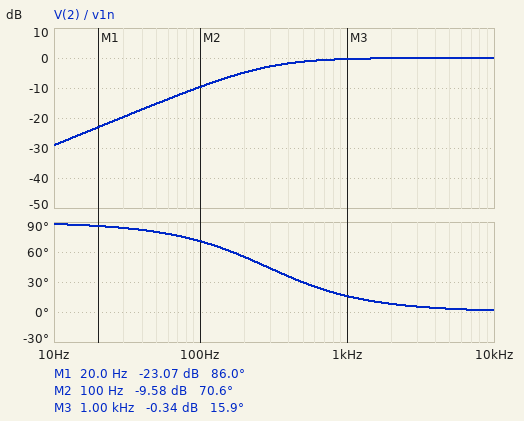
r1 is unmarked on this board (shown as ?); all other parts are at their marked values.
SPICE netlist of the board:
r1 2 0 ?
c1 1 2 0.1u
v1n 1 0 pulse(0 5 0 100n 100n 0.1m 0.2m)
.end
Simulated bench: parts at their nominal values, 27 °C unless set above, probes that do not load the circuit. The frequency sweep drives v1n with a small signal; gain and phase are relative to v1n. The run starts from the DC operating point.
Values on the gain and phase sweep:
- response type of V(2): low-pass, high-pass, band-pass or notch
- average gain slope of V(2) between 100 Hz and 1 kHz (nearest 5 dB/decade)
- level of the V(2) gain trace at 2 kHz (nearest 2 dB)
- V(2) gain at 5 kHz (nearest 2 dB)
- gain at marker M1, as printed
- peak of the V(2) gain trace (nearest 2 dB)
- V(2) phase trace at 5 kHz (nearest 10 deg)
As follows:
high-pass
10 dB/decade
0 dB
0 dB
-23.07 dB
0 dB
0 deg
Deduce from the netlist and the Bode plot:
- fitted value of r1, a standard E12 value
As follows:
5.6 kΩ
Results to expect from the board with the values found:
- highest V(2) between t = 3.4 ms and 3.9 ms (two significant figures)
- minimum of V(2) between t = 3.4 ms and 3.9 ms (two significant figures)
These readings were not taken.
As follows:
2.7 V
-2.7 V
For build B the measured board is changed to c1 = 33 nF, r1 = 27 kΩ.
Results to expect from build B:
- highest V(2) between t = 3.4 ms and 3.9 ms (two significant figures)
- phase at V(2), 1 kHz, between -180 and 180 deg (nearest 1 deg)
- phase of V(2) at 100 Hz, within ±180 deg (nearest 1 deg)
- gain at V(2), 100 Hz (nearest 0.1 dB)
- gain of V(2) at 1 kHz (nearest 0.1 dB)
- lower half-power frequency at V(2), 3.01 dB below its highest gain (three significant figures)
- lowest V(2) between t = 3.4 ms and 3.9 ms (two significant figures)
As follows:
2.7 V
10 deg
61 deg
-6.2 dB
-0.1 dB
179 Hz
-2.6 V
